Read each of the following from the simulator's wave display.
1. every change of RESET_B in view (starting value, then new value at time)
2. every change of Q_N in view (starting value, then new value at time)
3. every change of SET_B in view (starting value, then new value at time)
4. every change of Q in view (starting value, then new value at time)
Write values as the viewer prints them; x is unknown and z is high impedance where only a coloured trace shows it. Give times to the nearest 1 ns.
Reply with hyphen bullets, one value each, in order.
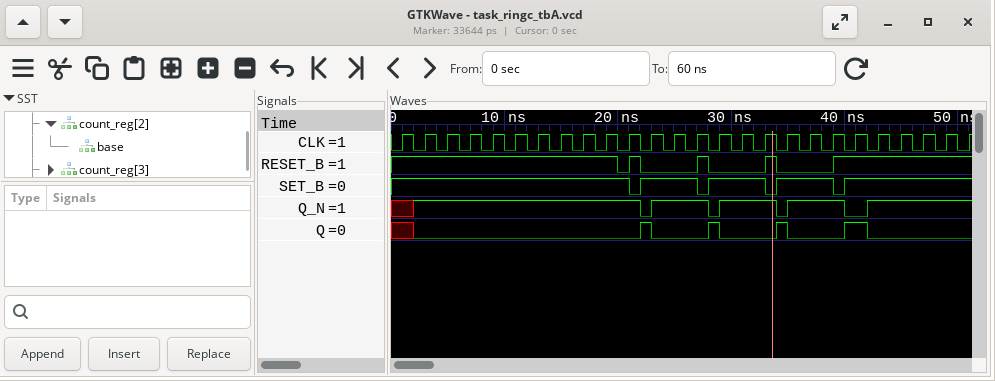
- 1, 0 at 20 ns, 1 at 21 ns, 0 at 22 ns, 1 at 27 ns, 0 at 28 ns, 1 at 33 ns, 0 at 34 ns, 1 at 39 ns
- x, 1 at 2 ns, 0 at 22 ns, 1 at 23 ns, 0 at 28 ns, 1 at 29 ns, 0 at 34 ns, 1 at 35 ns, 0 at 40 ns, 1 at 42 ns
- 1, 0 at 21 ns, 1 at 22 ns, 0 at 27 ns, 1 at 28 ns, 0 at 33 ns, 1 at 34 ns, 0 at 39 ns, 1 at 40 ns
- x, 0 at 2 ns, 1 at 22 ns, 0 at 23 ns, 1 at 28 ns, 0 at 29 ns, 1 at 34 ns, 0 at 35 ns, 1 at 40 ns, 0 at 42 ns
